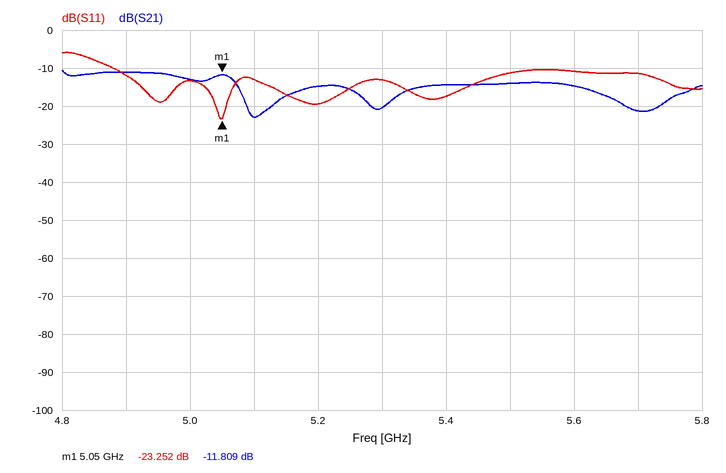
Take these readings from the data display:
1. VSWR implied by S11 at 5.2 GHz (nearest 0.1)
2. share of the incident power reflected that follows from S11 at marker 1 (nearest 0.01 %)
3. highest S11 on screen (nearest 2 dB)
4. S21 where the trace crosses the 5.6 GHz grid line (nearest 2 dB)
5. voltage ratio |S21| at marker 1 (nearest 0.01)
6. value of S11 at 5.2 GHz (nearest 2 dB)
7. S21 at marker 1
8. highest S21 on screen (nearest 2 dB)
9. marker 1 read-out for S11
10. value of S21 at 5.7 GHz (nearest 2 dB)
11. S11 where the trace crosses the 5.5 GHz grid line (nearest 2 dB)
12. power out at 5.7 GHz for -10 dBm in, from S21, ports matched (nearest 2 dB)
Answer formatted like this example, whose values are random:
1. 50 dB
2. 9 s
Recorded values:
1. 1.2
2. 0.47 %
3. -6 dB
4. -14 dB
5. 0.26
6. -20 dB
7. -11.809 dB
8. -10 dB
9. -23.252 dB
10. -22 dB
11. -12 dB
12. -32 dBm
